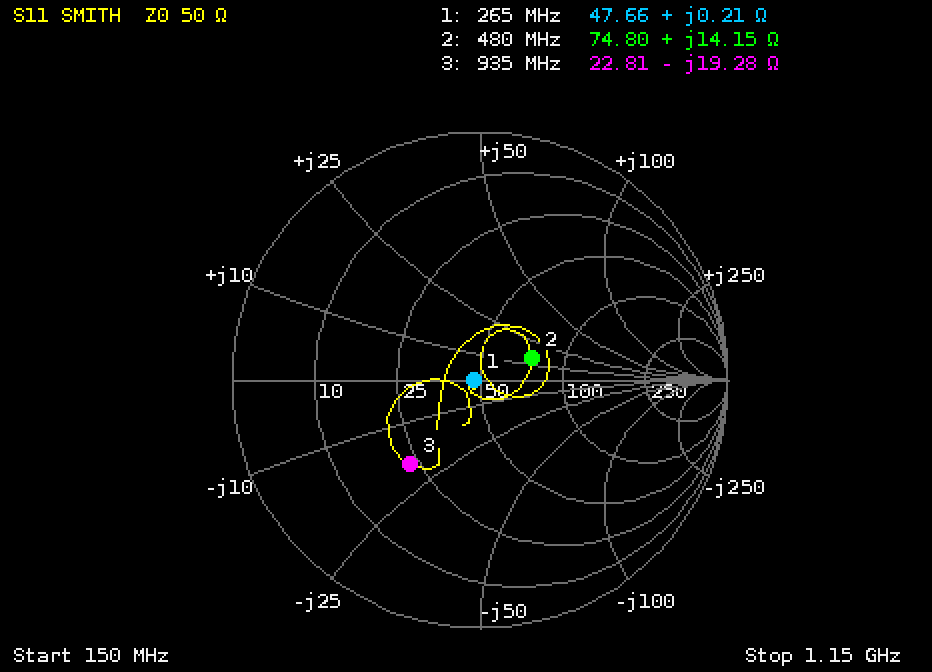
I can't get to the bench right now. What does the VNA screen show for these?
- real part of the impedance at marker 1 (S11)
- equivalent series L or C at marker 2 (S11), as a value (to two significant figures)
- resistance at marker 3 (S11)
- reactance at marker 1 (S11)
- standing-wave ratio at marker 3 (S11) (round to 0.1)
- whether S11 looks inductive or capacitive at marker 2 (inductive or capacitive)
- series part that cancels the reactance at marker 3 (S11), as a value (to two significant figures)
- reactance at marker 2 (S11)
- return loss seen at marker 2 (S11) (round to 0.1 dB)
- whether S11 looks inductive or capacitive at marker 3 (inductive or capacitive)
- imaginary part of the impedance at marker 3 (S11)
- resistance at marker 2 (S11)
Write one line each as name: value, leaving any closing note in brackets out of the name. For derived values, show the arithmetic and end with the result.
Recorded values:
real part of the impedance at marker 1: 47.66 Ω
equivalent series L or C at marker 2 (S11), as a value: L = 14.15 Ω/(2π × 480 MHz) ≈ 4.7 nH
resistance at marker 3: 22.81 Ω
reactance at marker 1: +0.21 Ω
standing-wave ratio at marker 3 (S11): 2.6
whether S11 looks inductive or capacitive at marker 2: inductive
series part that cancels the reactance at marker 3 (S11), as a value: L = 19.28 Ω/(2π × 935 MHz) ≈ 3.3 nH
reactance at marker 2: +14.15 Ω
return loss seen at marker 2 (S11): 12.9 dB
whether S11 looks inductive or capacitive at marker 3: capacitive
imaginary part of the impedance at marker 3: -19.28 Ω
resistance at marker 2: 74.80 Ω
